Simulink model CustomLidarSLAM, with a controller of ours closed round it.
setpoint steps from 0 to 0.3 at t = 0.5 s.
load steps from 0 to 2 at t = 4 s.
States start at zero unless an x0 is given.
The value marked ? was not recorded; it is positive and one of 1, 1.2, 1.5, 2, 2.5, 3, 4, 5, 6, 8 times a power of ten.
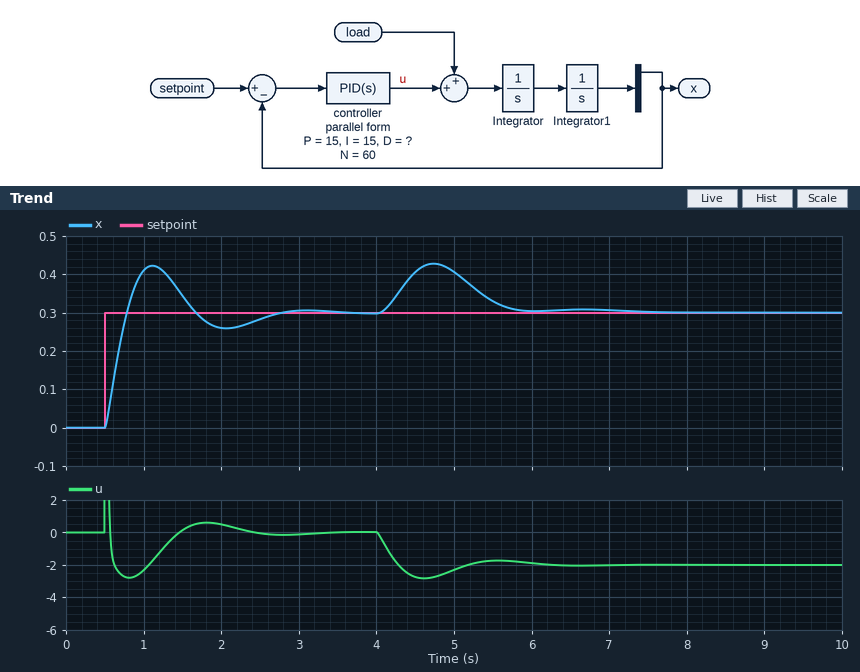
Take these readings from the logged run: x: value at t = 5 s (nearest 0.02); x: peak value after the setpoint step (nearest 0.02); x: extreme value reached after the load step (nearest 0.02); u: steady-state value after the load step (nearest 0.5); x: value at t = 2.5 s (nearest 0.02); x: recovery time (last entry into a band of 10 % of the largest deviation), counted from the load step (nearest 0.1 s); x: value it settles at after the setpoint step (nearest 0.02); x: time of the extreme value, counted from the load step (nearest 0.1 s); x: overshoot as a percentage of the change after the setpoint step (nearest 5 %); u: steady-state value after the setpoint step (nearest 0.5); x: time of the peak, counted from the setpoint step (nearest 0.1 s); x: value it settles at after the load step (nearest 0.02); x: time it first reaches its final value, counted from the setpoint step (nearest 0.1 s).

0.40
0.42
0.42
-2.0
0.28
1.7 s
0.30
0.7 s
40 %
0.0
0.6 s
0.30
0.3 s
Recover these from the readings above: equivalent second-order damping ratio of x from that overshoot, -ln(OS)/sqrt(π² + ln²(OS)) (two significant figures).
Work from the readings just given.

0.28
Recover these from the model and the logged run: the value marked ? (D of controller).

4
